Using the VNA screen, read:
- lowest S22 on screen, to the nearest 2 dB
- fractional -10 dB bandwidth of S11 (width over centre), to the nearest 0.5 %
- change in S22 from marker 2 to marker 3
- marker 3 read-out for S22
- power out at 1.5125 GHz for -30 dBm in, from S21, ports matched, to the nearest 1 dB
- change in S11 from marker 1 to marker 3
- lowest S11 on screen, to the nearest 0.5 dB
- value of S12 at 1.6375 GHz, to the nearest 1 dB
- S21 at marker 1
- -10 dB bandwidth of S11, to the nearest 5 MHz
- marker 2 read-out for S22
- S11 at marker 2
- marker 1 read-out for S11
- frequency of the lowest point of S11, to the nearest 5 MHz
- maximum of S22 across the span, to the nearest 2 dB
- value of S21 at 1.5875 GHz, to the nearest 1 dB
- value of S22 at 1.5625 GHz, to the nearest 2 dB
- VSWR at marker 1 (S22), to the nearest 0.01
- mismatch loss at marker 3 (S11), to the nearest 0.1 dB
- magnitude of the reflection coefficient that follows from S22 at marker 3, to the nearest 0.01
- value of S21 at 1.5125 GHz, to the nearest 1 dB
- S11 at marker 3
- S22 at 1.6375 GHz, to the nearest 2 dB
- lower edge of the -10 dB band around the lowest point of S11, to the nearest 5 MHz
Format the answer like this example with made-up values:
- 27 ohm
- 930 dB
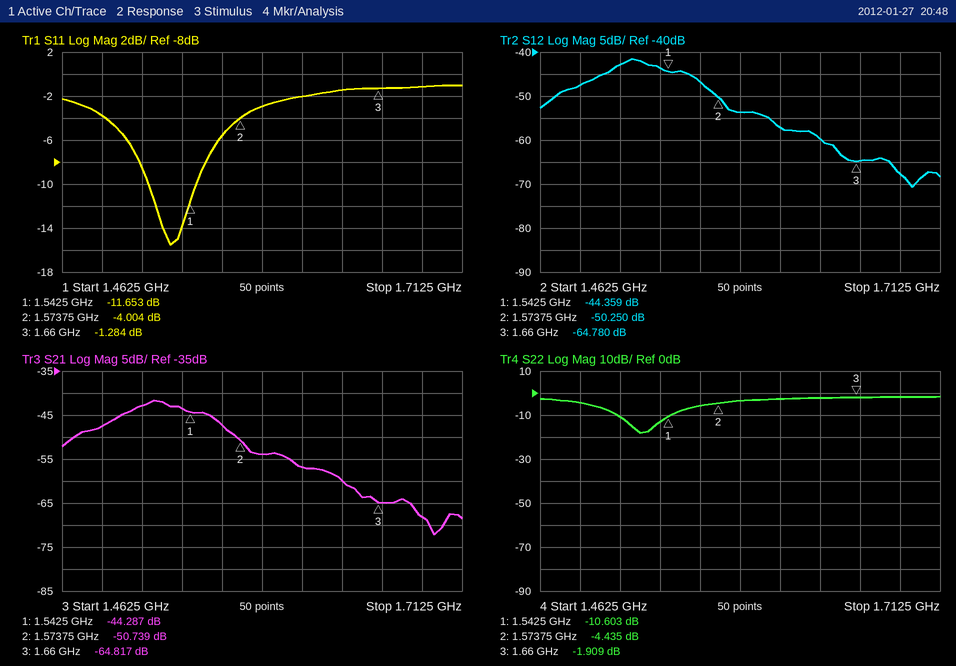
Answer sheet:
- -18 dB
- 2.0 %
- 2.526 dB
- -1.909 dB
- -73 dBm
- 10.369 dB
- -15.5 dB
- -60 dB
- -44.287 dB
- 30 MHz
- -4.435 dB
- -4.004 dB
- -11.653 dB
- 1.530 GHz
- -2 dB
- -54 dB
- -6 dB
- 1.84
- 5.9 dB
- 0.80
- -43 dB
- -1.284 dB
- -2 dB
- 1.515 GHz
